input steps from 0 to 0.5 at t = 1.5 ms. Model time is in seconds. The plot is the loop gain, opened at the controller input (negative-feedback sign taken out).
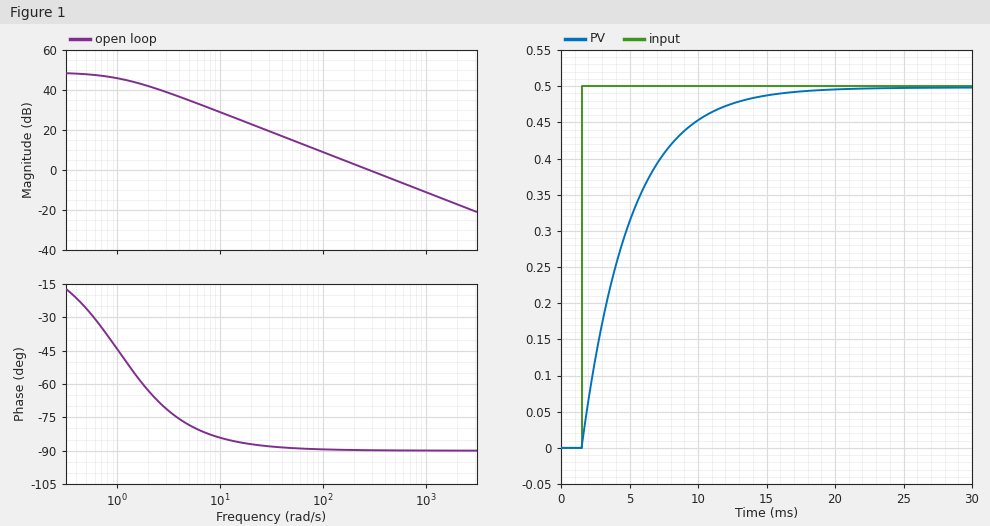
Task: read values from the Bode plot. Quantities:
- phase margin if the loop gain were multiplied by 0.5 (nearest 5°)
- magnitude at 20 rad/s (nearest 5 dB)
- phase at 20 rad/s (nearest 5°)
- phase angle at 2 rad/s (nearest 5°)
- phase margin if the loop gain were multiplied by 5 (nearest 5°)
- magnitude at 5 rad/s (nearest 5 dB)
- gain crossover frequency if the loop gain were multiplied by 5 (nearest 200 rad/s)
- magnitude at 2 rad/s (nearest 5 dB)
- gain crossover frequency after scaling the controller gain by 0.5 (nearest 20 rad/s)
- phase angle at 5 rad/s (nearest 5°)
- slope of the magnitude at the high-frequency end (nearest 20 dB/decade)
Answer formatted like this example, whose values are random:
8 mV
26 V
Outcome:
90°
25 dB
-85°
-65°
90°
35 dB
1400 rad/s
40 dB
140 rad/s
-80°
-20 dB/decade
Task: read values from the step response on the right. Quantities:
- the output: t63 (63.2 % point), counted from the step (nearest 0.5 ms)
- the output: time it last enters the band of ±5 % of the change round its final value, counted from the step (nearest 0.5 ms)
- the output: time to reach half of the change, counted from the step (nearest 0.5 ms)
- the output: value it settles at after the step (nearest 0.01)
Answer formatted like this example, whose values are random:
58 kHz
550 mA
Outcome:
3.5 ms
10.5 ms
2.5 ms
0.50
